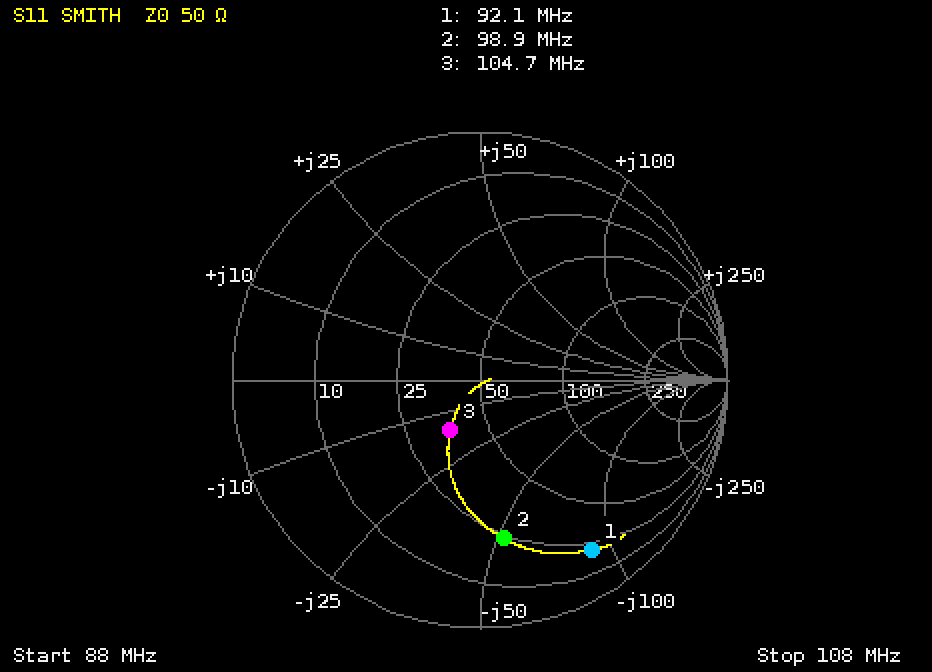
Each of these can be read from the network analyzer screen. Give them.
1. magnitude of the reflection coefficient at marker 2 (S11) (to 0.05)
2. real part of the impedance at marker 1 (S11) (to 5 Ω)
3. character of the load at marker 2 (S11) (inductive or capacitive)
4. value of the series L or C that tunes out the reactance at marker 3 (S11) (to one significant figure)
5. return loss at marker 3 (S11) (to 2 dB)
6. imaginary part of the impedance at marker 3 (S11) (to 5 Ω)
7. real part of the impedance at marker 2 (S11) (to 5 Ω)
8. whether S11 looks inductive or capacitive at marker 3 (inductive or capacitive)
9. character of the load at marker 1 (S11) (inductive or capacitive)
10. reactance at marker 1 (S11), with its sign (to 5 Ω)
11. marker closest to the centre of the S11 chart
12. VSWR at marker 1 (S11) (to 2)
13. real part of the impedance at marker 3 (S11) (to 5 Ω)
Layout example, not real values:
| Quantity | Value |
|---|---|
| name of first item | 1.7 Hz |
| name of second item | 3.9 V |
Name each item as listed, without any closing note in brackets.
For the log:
| Quantity | Value |
|---|---|
| magnitude of the reflection coefficient at marker 2 (S11) | 0.65 |
| real part of the impedance at marker 1 (S11) | 20 Ω |
| character of the load at marker 2 (S11) | capacitive |
| value of the series L or C that tunes out the reactance at marker 3 (S11) | 20 nH |
| return loss at marker 3 (S11) | 12 dB |
| imaginary part of the impedance at marker 3 (S11) | -15 Ω |
| real part of the impedance at marker 2 (S11) | 25 Ω |
| whether S11 looks inductive or capacitive at marker 3 | capacitive |
| character of the load at marker 1 (S11) | capacitive |
| reactance at marker 1 (S11), with its sign | -90 Ω |
| marker closest to the centre of the S11 chart | marker 3 |
| VSWR at marker 1 (S11) | 10 |
| real part of the impedance at marker 3 (S11) | 35 Ω |
